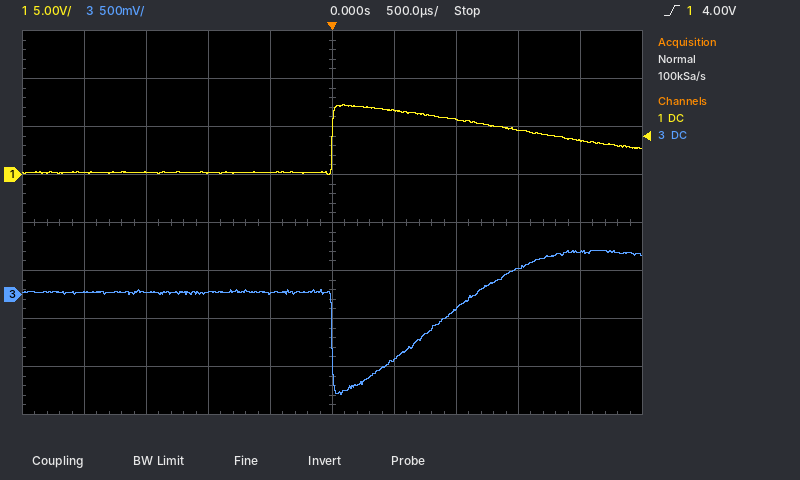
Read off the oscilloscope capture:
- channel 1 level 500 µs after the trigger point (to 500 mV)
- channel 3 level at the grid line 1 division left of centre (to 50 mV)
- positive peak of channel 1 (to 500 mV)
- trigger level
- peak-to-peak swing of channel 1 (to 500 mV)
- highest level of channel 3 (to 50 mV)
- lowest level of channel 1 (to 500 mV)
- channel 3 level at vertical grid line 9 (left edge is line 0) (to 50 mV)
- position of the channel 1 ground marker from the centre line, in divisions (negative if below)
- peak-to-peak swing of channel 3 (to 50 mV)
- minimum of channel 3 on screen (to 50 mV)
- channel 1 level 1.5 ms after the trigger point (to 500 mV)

6.5 V
0 mV
7.5 V
4.00 V
7.5 V
450 mV
0.0 V
450 mV
+1.0 div
1.50 V
-1.05 V
4.5 V
